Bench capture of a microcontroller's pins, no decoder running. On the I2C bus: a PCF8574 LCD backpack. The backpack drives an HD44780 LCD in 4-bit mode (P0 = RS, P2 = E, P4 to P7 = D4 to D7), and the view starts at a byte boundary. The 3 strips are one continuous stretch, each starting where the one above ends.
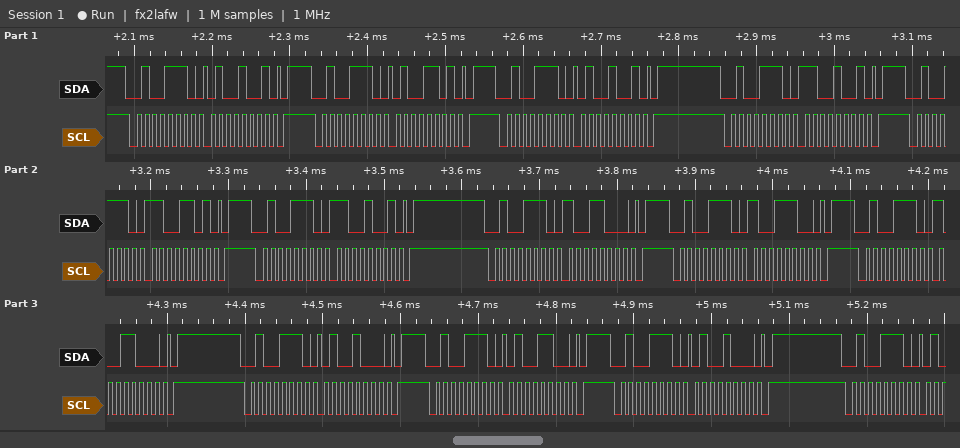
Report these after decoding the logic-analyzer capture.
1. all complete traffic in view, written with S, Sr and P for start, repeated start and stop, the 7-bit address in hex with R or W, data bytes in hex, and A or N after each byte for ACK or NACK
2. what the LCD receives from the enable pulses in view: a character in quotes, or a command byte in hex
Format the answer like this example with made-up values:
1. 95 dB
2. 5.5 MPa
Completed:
1. S 27W A 49 A P S 27W A 4D A P S 27W A 49 A P S 27W A C9 A P S 27W A CD A P S 27W A C9 A P S 27W A 98 A P S 27W A 9C A P S 27W A 98 A P S 27W A 48 A P S 27W A 4C A P S 27W A 48 A P S 27W A
2. 'L' 0x94
